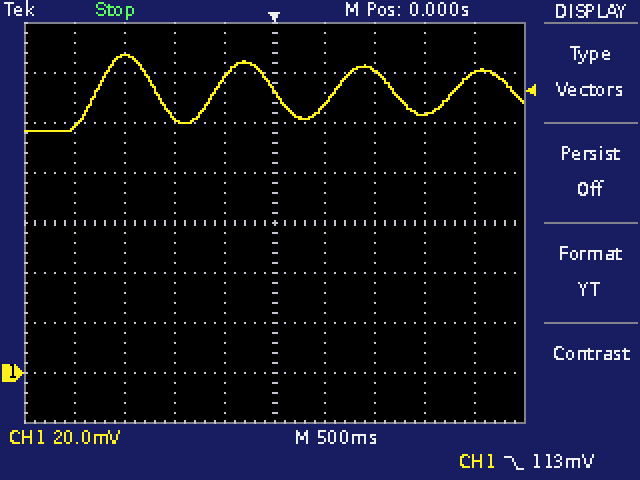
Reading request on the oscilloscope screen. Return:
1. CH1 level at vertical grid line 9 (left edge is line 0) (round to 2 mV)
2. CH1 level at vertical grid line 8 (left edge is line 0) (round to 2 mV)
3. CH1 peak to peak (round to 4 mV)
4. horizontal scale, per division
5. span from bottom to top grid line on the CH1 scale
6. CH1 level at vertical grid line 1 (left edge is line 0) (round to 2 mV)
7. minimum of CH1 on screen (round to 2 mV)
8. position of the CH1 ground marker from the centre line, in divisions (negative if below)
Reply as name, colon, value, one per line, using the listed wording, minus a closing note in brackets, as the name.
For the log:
CH1 level at vertical grid line 9 (left edge is line 0): 120 mV
CH1 level at vertical grid line 8 (left edge is line 0): 104 mV
CH1 peak to peak: 32 mV
horizontal scale, per division: 500 ms
span from bottom to top grid line on the CH1 scale: 160 mV
CH1 level at vertical grid line 1 (left edge is line 0): 98 mV
minimum of CH1 on screen: 96 mV
position of the CH1 ground marker from the centre line, in divisions: -3.0 div
